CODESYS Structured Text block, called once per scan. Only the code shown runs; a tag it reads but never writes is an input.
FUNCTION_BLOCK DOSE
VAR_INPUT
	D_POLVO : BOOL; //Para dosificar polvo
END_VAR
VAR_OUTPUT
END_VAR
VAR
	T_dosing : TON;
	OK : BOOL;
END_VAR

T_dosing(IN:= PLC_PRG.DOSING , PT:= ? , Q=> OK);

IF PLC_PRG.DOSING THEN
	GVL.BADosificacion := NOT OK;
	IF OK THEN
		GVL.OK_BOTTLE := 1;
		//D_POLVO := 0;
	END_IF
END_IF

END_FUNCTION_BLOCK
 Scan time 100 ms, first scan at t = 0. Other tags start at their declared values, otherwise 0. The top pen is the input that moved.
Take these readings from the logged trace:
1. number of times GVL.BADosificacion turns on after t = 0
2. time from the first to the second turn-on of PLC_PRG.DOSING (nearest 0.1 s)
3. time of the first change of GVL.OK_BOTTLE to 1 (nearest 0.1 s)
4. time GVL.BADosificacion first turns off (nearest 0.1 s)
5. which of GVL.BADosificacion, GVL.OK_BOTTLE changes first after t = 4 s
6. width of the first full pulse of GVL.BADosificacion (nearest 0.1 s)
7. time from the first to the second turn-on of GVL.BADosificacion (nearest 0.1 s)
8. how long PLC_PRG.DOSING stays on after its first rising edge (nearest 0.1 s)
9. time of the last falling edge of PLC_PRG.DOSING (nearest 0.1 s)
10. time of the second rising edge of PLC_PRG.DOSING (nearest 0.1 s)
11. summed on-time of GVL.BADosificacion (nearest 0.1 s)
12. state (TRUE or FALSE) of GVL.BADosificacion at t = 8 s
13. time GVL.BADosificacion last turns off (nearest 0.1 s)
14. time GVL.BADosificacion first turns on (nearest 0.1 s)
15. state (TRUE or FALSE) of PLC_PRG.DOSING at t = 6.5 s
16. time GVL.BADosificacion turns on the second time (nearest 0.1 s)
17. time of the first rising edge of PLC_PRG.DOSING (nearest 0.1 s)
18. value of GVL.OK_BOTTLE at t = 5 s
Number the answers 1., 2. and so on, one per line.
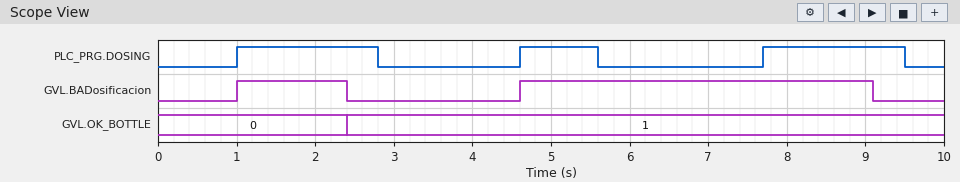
1. 2
2. 3.6 s
3. 2.4 s
4. 2.4 s
5. GVL.BADosificacion
6. 1.4 s
7. 3.6 s
8. 1.8 s
9. 9.5 s
10. 4.6 s
11. 5.9 s
12. TRUE
13. 9.1 s
14. 1.0 s
15. FALSE
16. 4.6 s
17. 1.0 s
18. 1
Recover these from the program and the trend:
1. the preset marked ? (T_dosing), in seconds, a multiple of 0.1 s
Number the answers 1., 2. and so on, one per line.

1. 1.4 s
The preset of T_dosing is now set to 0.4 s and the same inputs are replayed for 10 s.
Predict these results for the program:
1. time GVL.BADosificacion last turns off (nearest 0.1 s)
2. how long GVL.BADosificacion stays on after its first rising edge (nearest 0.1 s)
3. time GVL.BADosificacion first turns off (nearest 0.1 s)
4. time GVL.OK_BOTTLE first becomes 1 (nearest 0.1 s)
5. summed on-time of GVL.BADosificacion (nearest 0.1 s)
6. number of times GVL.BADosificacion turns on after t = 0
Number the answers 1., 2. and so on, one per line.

1. 8.1 s
2. 0.4 s
3. 1.4 s
4. 1.4 s
5. 1.2 s
6. 3
